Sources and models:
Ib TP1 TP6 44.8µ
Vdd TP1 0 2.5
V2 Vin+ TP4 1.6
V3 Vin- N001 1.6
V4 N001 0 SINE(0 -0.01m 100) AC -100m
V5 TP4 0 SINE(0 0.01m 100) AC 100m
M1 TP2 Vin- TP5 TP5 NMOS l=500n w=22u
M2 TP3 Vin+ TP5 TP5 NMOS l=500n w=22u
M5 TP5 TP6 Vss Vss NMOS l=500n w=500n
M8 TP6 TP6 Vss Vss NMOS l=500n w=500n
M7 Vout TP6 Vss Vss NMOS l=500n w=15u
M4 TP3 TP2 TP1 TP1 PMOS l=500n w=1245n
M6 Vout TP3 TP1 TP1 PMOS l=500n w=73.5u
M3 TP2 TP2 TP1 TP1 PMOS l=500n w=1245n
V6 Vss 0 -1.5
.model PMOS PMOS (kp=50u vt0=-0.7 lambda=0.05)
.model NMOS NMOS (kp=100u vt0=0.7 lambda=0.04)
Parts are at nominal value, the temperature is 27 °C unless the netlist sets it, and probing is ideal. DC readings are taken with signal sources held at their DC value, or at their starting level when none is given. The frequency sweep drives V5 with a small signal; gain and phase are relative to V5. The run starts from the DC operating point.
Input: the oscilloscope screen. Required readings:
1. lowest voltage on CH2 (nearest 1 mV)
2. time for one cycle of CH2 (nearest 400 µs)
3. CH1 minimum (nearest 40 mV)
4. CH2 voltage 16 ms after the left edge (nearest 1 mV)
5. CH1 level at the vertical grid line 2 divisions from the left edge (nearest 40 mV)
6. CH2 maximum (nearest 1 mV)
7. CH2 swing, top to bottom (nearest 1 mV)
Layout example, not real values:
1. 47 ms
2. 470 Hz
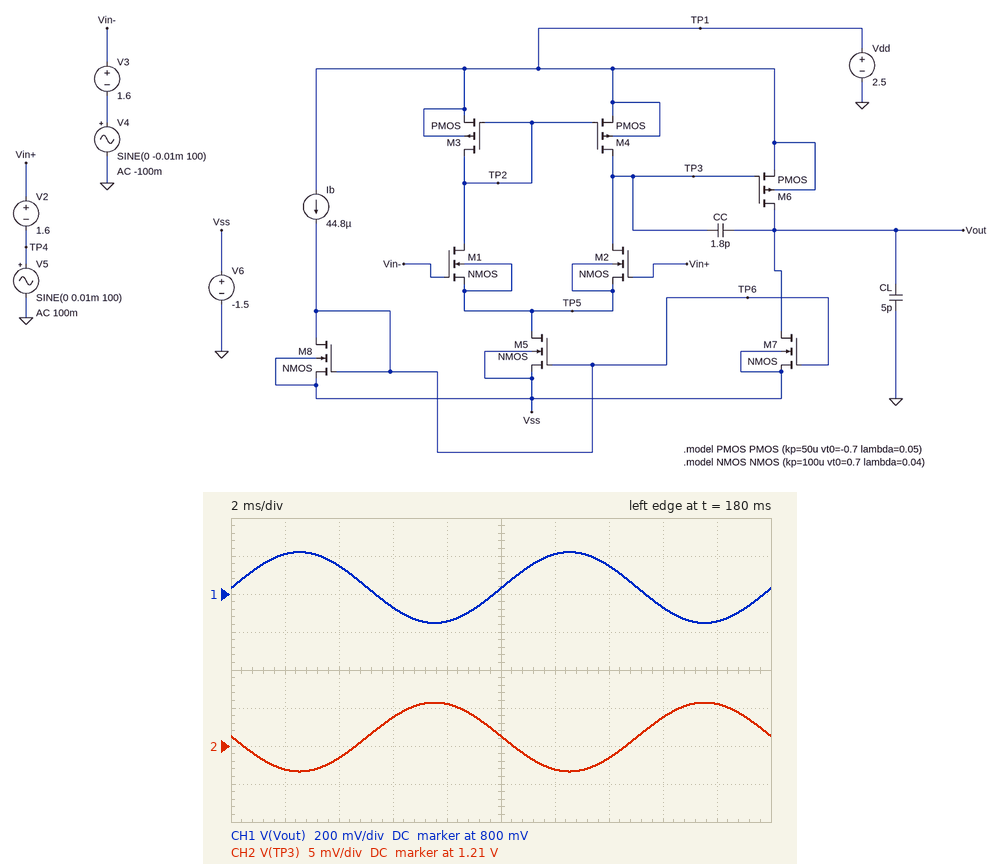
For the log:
1. 1.207 V
2. 10.0 ms
3. 640 mV
4. 1.214 V
5. 960 mV
6. 1.216 V
7. 9 mV
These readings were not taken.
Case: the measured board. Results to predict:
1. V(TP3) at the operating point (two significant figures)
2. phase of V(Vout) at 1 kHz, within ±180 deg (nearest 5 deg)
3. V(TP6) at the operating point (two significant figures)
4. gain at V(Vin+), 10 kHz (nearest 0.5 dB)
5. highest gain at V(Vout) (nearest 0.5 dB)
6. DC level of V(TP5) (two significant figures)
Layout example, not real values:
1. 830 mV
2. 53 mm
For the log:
1. 1.2 V
2. -15 deg
3. 120 mV
4. 0 dB
5. 80.0 dB
6. 800 mV
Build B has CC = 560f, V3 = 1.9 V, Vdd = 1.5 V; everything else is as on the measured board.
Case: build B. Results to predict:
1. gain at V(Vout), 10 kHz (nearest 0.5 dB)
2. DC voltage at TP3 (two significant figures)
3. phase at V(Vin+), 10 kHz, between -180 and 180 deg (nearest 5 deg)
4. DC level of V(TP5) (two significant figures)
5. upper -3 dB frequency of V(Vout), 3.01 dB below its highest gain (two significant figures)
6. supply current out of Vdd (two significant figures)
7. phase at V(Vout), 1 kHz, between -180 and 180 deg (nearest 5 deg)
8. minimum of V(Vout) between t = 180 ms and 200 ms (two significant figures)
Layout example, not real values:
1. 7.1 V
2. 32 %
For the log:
1. -6.5 dB
2. 220 mV
3. 0 deg
4. 210 mV
5. 780 kHz
6. 1.4 mA
7. 0 deg
8. -69 mV
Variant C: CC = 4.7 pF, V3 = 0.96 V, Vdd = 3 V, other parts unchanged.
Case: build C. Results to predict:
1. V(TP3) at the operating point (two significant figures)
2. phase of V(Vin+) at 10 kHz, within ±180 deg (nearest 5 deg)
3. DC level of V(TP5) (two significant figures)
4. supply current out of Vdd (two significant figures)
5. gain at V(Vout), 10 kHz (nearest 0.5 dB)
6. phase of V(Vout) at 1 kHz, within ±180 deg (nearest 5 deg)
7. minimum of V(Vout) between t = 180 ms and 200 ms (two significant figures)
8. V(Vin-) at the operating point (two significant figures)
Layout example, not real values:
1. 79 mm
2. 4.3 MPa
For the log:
1. 170 mV
2. 0 deg
3. 160 mV
4. 1.6 mA
5. -45.5 dB
6. 0 deg
7. 2.9 V
8. 960 mV
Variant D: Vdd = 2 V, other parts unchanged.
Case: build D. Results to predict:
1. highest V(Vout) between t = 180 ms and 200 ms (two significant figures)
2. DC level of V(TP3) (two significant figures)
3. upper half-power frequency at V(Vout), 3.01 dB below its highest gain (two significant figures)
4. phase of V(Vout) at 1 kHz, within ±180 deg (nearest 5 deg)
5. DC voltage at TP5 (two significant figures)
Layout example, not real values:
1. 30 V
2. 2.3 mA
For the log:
1. 510 mV
2. 710 mV
3. 260 kHz
4. 0 deg
5. 690 mV
